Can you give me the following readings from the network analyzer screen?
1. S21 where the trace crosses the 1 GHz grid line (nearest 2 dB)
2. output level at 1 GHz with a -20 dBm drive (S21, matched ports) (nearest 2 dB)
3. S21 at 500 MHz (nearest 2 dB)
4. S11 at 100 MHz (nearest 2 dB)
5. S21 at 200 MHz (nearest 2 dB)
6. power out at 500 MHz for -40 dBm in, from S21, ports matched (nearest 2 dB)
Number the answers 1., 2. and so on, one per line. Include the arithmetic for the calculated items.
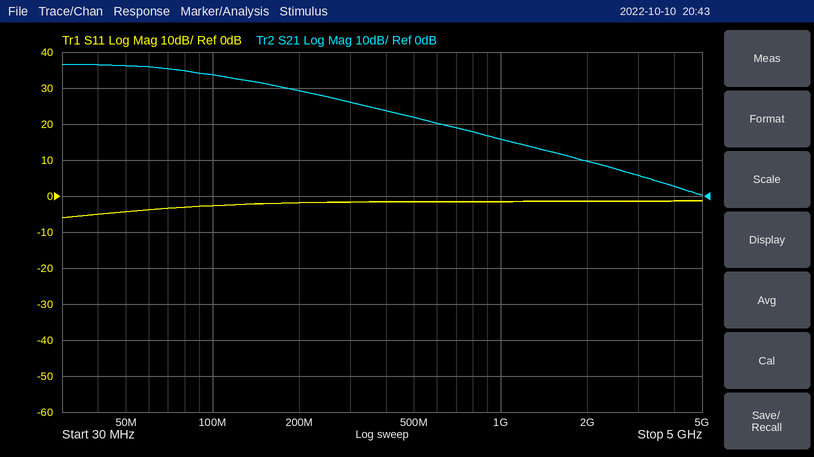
1. 16 dB
2. -20 dBm + (16 dB) = -4 dBm
3. 22 dB
4. -2 dB
5. 30 dB
6. -40 dBm + (22 dB) = -18 dBm
